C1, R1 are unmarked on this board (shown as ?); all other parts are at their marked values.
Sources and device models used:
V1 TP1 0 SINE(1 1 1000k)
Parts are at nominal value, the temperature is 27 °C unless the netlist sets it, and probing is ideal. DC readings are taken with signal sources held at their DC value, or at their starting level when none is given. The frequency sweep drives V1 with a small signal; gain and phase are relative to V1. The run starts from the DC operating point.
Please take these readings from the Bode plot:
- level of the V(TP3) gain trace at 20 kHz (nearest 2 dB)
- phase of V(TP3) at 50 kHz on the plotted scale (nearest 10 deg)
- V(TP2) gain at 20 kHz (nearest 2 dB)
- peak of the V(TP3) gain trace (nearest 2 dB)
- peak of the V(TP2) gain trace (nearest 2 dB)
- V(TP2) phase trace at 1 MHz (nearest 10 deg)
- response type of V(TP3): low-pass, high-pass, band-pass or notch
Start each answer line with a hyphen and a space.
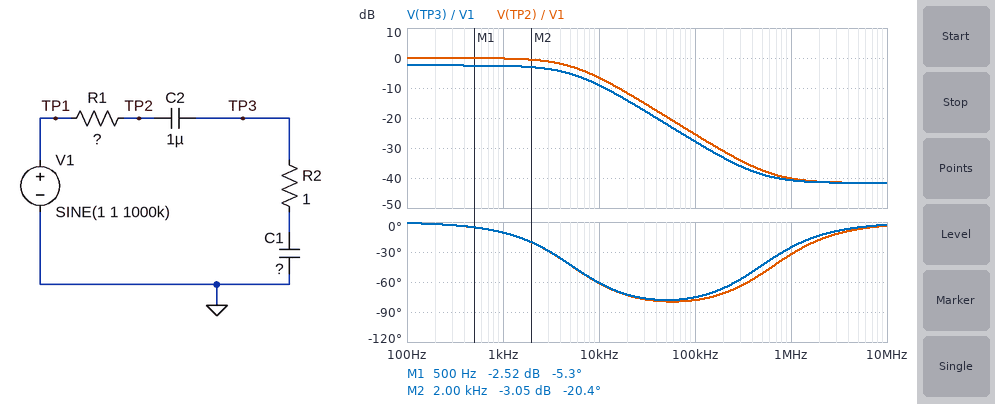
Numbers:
- -14 dB
- -80 deg
- -12 dB
- -2 dB
- 0 dB
- -30 deg
- low-pass
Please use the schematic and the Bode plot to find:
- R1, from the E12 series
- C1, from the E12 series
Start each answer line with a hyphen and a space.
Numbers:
- 120 Ω
- 330 nF
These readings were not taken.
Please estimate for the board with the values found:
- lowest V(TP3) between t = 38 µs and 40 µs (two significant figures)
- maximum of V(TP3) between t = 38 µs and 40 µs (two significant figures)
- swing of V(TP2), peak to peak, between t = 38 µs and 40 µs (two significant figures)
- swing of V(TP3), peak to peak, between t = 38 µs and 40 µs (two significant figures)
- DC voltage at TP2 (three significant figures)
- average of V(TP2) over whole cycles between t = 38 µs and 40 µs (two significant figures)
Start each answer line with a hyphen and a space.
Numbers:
- -8.1 mV
- 10 mV
- 20 mV
- 18 mV
- 1.00 V
- 1.0 V
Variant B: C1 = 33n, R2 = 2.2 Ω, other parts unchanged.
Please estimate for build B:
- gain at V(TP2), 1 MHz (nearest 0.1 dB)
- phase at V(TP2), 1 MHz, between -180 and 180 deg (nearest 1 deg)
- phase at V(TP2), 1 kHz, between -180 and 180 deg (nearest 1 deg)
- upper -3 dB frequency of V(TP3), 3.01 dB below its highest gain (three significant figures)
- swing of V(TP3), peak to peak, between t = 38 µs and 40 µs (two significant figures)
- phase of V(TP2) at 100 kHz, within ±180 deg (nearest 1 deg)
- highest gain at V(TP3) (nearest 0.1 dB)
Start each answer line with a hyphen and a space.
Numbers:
- -27.0 dB
- -64 deg
- -1 deg
- 40.8 kHz
- 87 mV
- -65 deg
- -0.3 dB
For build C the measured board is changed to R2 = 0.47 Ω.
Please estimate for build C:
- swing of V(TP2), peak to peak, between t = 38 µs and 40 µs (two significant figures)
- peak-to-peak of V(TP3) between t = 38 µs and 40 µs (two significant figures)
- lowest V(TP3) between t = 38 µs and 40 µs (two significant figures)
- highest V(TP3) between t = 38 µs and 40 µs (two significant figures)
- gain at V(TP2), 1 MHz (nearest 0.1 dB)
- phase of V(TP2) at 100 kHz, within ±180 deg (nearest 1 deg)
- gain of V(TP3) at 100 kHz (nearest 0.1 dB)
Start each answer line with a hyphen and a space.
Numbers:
- 13 mV
- 11 mV
- -4.5 mV
- 6.7 mV
- -43.6 dB
- -83 deg
- -27.9 dB
